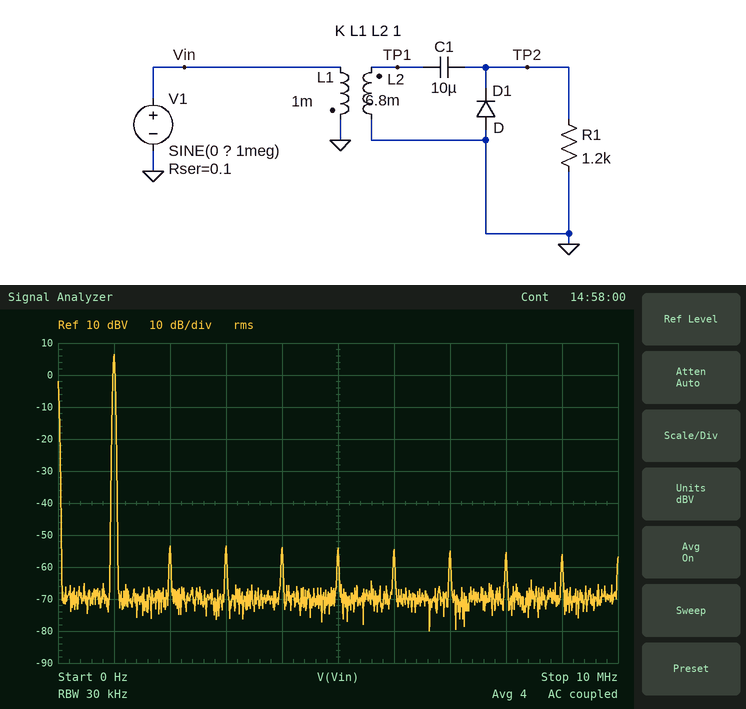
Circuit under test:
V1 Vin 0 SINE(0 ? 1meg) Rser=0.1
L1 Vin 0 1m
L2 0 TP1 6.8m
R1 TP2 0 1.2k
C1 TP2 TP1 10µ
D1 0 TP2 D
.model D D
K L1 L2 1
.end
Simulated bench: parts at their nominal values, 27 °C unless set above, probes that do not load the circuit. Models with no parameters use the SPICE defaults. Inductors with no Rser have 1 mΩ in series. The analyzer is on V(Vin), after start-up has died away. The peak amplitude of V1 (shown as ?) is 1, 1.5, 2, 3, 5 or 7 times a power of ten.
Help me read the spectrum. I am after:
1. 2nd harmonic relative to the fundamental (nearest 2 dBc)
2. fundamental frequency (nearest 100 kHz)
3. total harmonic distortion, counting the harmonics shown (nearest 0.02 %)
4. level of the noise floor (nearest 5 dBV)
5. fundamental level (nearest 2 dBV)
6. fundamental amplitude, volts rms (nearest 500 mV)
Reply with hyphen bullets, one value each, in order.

- -60 dBc
- 1.0 MHz
- 0.10 %
- -70 dBV
- 6 dBV
- 2.0 V
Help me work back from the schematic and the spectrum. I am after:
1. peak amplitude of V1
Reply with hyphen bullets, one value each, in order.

- 3 V
